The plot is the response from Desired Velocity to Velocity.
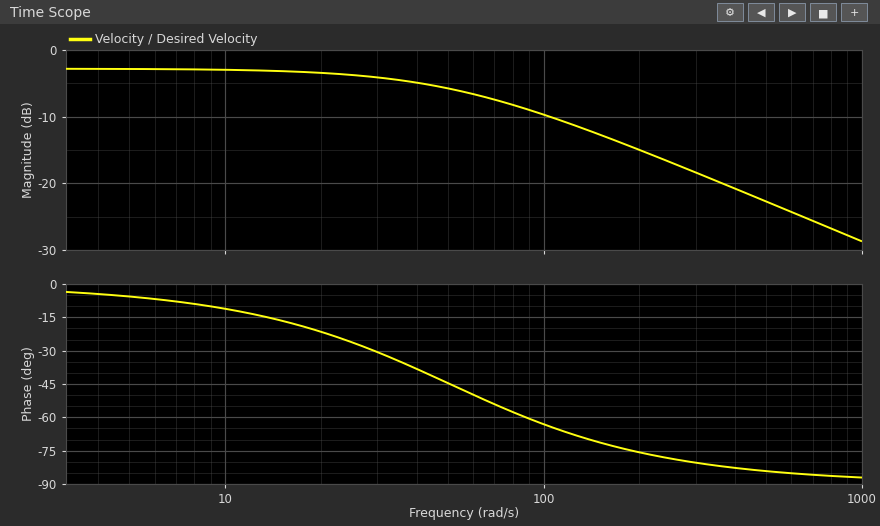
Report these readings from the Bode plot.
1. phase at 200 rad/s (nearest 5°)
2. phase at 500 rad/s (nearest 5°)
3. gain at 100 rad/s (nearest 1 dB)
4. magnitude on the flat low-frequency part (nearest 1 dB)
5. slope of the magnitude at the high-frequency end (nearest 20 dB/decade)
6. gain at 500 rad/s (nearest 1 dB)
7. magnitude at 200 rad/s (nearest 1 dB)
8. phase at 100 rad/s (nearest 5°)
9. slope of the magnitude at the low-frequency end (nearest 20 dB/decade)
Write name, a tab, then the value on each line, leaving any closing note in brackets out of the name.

phase at 200 rad/s	-75°
phase at 500 rad/s	-85°
gain at 100 rad/s	-10 dB
magnitude on the flat low-frequency part	-3 dB
slope of the magnitude at the high-frequency end	-20 dB/decade
gain at 500 rad/s	-23 dB
magnitude at 200 rad/s	-15 dB
phase at 100 rad/s	-65°
slope of the magnitude at the low-frequency end	0 dB/decade
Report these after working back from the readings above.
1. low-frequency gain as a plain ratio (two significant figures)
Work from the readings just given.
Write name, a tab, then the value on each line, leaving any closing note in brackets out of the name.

low-frequency gain as a plain ratio	0.71
